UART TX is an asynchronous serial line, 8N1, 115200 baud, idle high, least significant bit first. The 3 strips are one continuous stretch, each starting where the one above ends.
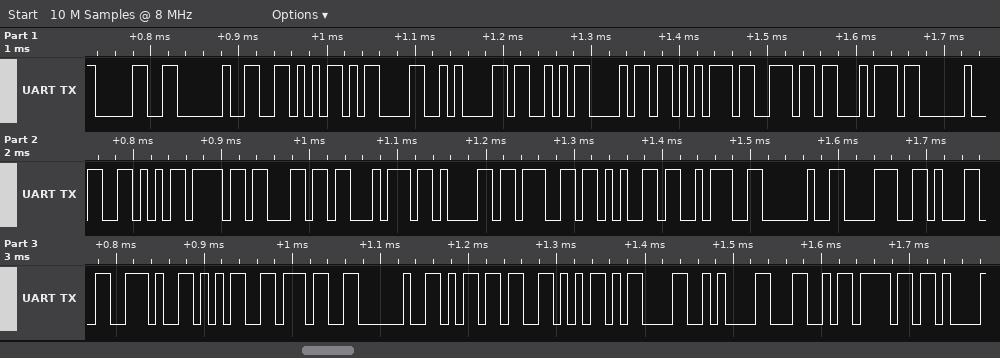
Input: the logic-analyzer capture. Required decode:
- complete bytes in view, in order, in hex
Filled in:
30 20 56 0D 0A 53 68 75 6E 74 20 56 6F 6C 74 61 67 65 3A 20 38 31 2E 35 37 20 6D 56 0D 0A 4C 6F
